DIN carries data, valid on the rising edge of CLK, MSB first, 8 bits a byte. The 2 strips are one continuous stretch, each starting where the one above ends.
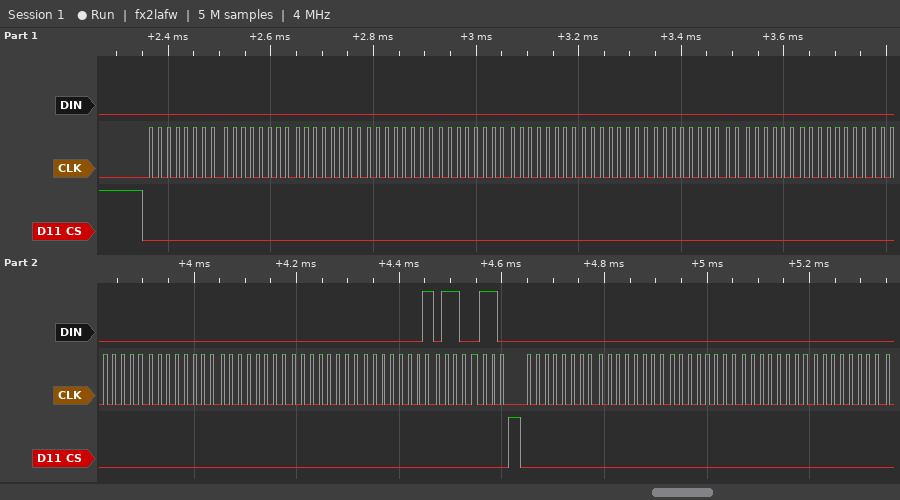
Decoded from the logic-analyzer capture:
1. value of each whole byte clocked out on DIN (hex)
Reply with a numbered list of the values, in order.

1. 00 00 00 00 00 00 00 00 00 00 00 00 00 00 01 66 00 00 00 00 00
